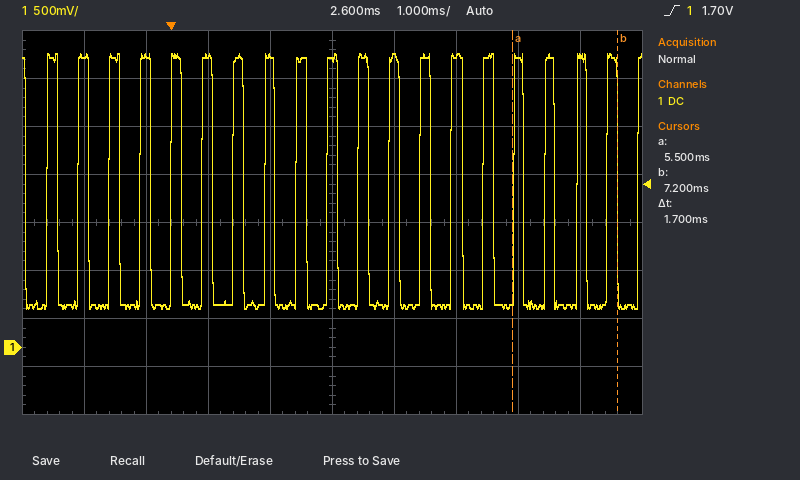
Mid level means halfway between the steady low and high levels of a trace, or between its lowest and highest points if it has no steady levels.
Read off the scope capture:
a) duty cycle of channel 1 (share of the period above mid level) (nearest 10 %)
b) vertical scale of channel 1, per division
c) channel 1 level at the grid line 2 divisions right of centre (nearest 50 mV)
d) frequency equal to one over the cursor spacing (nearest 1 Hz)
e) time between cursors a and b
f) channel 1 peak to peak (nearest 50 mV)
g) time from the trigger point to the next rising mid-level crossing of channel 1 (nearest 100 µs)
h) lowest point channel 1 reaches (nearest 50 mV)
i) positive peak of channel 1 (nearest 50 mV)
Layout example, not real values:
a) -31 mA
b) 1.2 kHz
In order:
a) 30 %
b) 500 mV
c) 3.05 V
d) 588 Hz
e) 1.7 ms
f) 2.65 V
g) 500 µs
h) 400 mV
i) 3.05 V
